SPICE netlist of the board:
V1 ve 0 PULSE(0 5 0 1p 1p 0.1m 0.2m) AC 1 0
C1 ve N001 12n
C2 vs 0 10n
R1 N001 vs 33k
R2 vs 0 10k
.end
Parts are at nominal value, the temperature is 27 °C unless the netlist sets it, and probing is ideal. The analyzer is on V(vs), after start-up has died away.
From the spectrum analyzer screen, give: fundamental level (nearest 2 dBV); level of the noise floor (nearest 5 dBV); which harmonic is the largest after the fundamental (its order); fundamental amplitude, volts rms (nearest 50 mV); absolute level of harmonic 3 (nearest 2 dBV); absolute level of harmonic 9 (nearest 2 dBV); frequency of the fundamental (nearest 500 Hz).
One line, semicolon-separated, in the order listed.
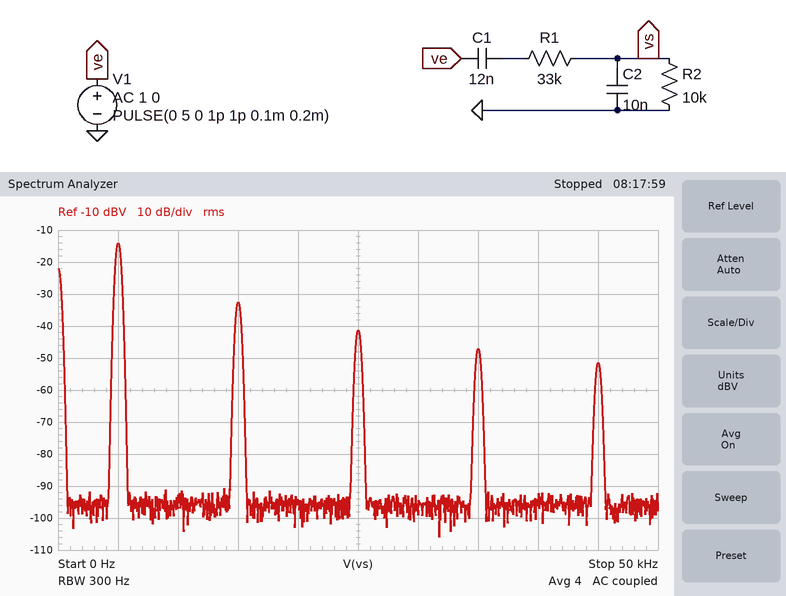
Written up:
-14 dBV; -95 dBV; 3; 200 mV; -32 dBV; -52 dBV; 5.0 kHz
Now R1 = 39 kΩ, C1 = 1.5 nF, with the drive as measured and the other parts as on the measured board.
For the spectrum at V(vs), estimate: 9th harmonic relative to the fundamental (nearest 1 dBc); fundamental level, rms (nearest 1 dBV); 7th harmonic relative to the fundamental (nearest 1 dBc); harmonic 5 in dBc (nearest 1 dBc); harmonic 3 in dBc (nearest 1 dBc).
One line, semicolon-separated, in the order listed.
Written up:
-36 dBc; -17 dBV; -32 dBc; -26 dBc; -17 dBc
